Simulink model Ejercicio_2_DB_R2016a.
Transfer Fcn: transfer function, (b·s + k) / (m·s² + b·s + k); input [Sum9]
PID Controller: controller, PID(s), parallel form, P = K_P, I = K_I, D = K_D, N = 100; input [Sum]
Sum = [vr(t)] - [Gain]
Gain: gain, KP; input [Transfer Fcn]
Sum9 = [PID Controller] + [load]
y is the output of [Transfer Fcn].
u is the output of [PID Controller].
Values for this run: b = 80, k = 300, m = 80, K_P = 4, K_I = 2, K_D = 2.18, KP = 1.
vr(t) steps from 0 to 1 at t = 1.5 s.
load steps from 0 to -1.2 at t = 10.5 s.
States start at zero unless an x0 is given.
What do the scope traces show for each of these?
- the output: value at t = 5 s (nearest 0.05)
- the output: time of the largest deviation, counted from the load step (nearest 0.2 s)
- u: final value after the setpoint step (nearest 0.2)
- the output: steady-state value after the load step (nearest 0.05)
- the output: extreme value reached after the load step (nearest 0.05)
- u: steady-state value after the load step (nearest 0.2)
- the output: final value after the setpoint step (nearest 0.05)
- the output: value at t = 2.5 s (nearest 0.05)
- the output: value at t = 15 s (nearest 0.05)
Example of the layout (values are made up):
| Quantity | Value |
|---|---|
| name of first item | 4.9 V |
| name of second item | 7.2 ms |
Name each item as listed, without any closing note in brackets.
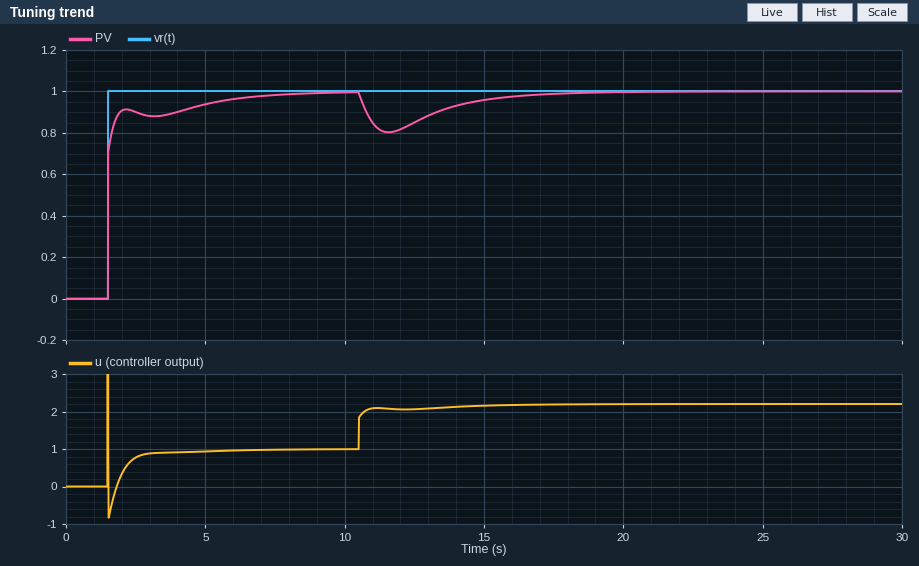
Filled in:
| Quantity | Value |
|---|---|
| the output: value at t = 5 s | 0.95 |
| the output: time of the largest deviation, counted from the load step | 1.0 s |
| u: final value after the setpoint step | 1.0 |
| the output: steady-state value after the load step | 1.00 |
| the output: extreme value reached after the load step | 0.80 |
| u: steady-state value after the load step | 2.2 |
| the output: final value after the setpoint step | 1.00 |
| the output: value at t = 2.5 s | 0.90 |
| the output: value at t = 15 s | 0.95 |
